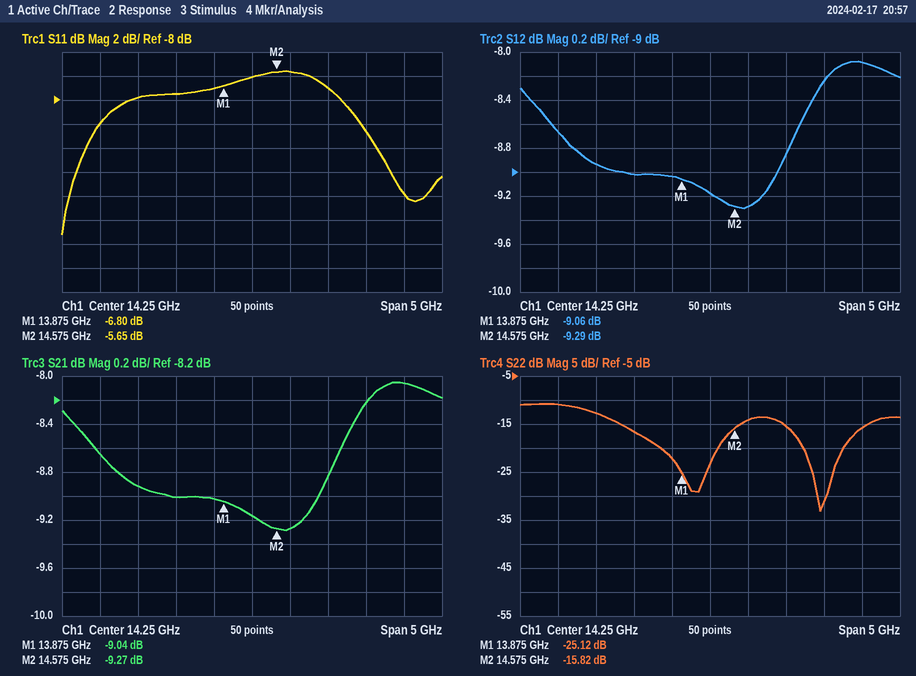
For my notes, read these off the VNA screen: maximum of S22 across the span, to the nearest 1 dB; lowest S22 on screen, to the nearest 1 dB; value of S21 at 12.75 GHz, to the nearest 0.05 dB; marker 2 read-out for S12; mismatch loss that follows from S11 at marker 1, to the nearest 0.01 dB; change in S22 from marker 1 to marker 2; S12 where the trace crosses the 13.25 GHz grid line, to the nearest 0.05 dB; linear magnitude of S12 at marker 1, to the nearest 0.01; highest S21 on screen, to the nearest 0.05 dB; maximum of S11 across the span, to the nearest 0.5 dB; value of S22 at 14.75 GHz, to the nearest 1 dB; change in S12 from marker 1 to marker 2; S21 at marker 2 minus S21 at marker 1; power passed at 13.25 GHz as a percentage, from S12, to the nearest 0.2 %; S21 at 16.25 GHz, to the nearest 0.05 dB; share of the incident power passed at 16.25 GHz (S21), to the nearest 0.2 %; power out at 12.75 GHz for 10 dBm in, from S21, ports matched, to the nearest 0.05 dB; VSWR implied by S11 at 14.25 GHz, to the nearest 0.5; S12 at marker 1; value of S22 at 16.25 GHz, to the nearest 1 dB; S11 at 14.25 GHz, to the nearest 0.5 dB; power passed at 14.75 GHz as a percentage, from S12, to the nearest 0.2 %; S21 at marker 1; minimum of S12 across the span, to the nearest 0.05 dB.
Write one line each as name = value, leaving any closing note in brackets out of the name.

maximum of S22 across the span, to the nearest 1 dB = -11 dB
lowest S22 on screen, to the nearest 1 dB = -33 dB
value of S21 at 12.75 GHz, to the nearest 0.05 dB = -8.90 dB
marker 2 read-out for S12 = -9.29 dB
mismatch loss that follows from S11 at marker 1, to the nearest 0.01 dB = 1.02 dB
change in S22 from marker 1 to marker 2 = 9.30 dB
S12 where the trace crosses the 13.25 GHz grid line, to the nearest 0.05 dB = -9.00 dB
linear magnitude of S12 at marker 1, to the nearest 0.01 = 0.35
highest S21 on screen, to the nearest 0.05 dB = -8.05 dB
maximum of S11 across the span, to the nearest 0.5 dB = -5.5 dB
value of S22 at 14.75 GHz, to the nearest 1 dB = -14 dB
change in S12 from marker 1 to marker 2 = -0.23 dB
S21 at marker 2 minus S21 at marker 1 = -0.23 dB
power passed at 13.25 GHz as a percentage, from S12, to the nearest 0.2 % = 12.6 %
S21 at 16.25 GHz, to the nearest 0.05 dB = -8.05 dB
share of the incident power passed at 16.25 GHz (S21), to the nearest 0.2 % = 15.6 %
power out at 12.75 GHz for 10 dBm in, from S21, ports matched, to the nearest 0.05 dB = 1.10 dBm
VSWR implied by S11 at 14.25 GHz, to the nearest 0.5 = 3.0
S12 at marker 1 = -9.06 dB
value of S22 at 16.25 GHz, to the nearest 1 dB = -16 dB
S11 at 14.25 GHz, to the nearest 0.5 dB = -6.0 dB
power passed at 14.75 GHz as a percentage, from S12, to the nearest 0.2 % = 11.8 %
S21 at marker 1 = -9.04 dB
minimum of S12 across the span, to the nearest 0.05 dB = -9.30 dB
